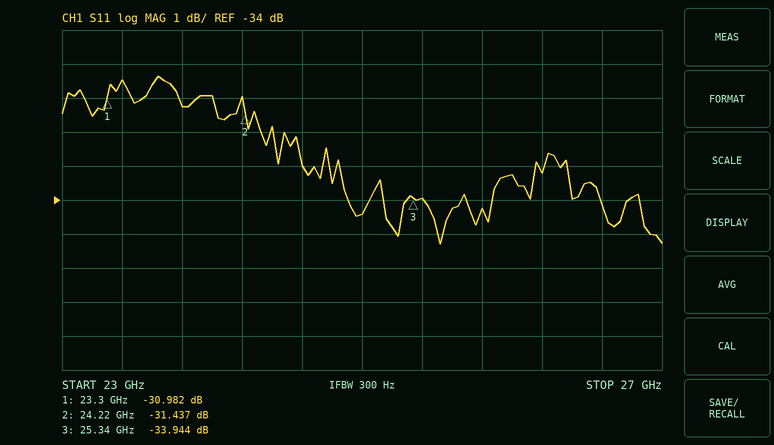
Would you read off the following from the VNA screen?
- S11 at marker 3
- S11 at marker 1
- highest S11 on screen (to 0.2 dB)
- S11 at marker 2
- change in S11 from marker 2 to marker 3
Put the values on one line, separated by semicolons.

-33.944 dB; -30.982 dB; -30.4 dB; -31.437 dB; -2.507 dB
